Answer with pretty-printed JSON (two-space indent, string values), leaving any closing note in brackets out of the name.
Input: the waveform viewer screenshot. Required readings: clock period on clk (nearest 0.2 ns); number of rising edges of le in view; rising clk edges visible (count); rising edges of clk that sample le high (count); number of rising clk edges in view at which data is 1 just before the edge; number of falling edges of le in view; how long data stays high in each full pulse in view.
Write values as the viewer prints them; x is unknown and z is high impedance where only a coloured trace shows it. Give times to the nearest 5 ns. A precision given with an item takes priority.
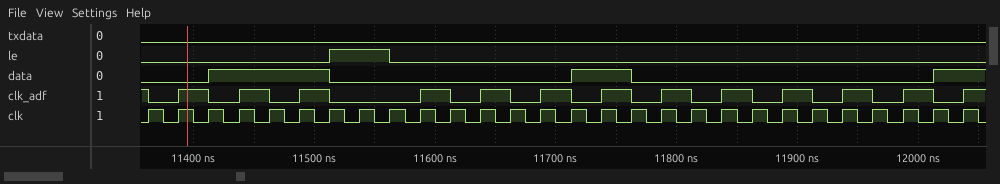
{
  "clock period on clk": "25 ns",
  "number of rising edges of le in view": "1",
  "rising clk edges visible": "28",
  "rising edges of clk that sample le high": "2",
  "number of rising clk edges in view at which data is 1 just before the edge": "7",
  "number of falling edges of le in view": "1",
  "how long data stays high in each full pulse in view": "100 ns, 50 ns"
}
